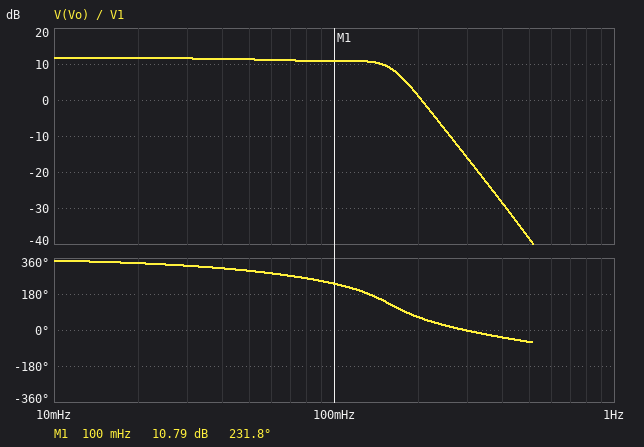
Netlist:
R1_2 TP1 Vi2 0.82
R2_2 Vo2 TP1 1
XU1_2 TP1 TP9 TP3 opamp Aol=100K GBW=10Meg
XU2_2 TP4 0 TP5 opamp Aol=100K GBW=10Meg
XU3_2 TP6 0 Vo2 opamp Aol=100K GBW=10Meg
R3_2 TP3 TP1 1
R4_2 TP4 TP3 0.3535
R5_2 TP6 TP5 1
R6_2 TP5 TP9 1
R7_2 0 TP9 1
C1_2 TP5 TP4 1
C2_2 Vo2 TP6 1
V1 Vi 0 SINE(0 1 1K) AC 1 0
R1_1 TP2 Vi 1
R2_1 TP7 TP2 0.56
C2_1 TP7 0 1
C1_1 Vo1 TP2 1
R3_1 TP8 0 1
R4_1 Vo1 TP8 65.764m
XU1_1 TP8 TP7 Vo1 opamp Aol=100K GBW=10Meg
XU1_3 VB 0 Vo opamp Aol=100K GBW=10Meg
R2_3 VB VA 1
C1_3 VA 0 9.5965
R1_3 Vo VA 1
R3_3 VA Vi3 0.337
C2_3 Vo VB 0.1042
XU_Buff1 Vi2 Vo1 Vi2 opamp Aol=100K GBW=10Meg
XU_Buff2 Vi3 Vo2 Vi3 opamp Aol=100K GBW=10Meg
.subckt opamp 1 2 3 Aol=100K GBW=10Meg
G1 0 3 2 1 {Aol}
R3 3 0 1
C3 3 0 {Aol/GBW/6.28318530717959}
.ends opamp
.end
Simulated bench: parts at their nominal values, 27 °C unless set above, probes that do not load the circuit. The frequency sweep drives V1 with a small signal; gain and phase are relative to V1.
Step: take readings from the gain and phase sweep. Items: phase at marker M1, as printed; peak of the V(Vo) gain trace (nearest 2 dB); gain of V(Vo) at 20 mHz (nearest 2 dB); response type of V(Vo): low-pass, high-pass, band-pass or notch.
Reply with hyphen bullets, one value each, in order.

- 231.8 deg
- 12 dB
- 12 dB
- low-pass
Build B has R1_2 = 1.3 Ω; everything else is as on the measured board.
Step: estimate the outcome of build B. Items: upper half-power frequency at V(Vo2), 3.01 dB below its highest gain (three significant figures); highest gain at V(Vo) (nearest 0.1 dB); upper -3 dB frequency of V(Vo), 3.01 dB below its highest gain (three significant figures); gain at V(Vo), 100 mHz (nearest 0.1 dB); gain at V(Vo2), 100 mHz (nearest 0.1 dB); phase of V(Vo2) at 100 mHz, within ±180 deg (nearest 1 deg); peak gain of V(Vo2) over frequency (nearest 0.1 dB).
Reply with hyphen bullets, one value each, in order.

- 92.2 mHz
- 7.7 dB
- 167 mHz
- 7.5 dB
- -5.2 dB
- 84 deg
- -1.7 dB
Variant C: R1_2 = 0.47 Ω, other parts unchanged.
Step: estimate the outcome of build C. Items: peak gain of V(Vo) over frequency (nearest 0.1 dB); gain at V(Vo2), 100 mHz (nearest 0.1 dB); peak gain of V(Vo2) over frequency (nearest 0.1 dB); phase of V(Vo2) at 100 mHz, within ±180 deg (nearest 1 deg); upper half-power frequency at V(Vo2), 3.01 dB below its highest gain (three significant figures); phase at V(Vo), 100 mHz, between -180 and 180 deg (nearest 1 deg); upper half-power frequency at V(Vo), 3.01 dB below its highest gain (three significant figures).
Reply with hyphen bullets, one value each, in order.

- 16.6 dB
- 1.5 dB
- 7.1 dB
- 73 deg
- 67.8 mHz
- -135 deg
- 139 mHz
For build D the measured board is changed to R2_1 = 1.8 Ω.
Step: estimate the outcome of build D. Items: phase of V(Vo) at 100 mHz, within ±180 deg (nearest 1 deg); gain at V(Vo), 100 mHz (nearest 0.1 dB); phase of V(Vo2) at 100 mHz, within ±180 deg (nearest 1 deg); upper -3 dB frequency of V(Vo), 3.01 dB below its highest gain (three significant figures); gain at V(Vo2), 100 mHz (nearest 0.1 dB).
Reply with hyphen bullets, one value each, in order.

- -158 deg
- 7.7 dB
- 50 deg
- 78.7 mHz
- -5.0 dB
